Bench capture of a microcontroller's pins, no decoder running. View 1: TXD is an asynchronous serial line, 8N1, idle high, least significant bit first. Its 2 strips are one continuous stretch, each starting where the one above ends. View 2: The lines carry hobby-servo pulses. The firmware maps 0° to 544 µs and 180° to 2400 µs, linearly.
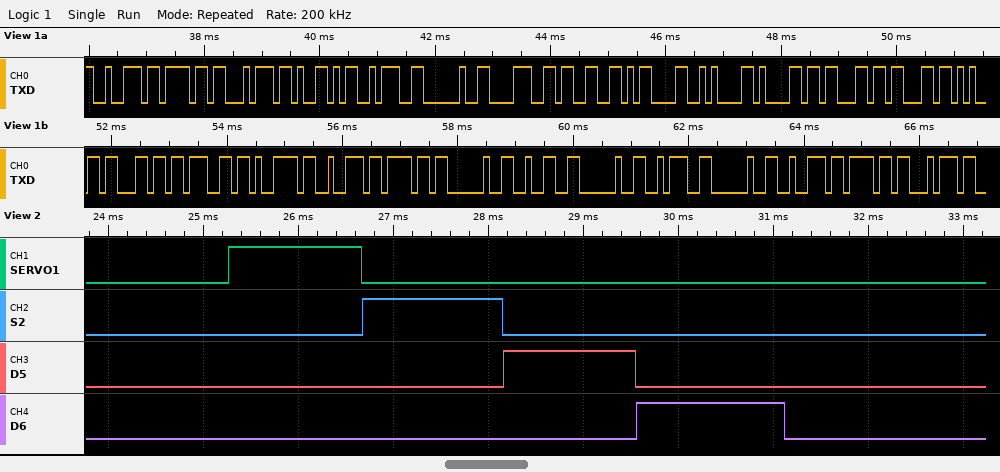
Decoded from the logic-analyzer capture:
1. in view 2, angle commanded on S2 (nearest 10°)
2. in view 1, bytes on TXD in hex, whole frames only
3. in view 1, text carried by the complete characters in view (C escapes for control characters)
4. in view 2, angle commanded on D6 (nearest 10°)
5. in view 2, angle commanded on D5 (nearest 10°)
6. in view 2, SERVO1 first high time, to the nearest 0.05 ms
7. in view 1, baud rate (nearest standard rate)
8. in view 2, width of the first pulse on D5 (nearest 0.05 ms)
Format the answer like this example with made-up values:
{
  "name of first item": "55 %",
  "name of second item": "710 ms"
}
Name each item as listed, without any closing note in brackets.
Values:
{
  "in view 2, angle commanded on S2": "90°",
  "in view 1, bytes on TXD in hex, whole frames only": "72 6F 74 59 3A 20 38 33 0D 0A 61 63 63 65 6C 67 79 72 6F 20 32 20 3A 20 72 6F 74",
  "in view 1, text carried by the complete characters in view": "\"rotY: 83\\r\\naccelgyro 2 : rot\"",
  "in view 2, angle commanded on D6": "100°",
  "in view 2, angle commanded on D5": "80°",
  "in view 2, SERVO1 first high time, to the nearest 0.05 ms": "1.40 ms",
  "in view 1, baud rate": "9600 baud",
  "in view 2, width of the first pulse on D5": "1.40 ms"
}
